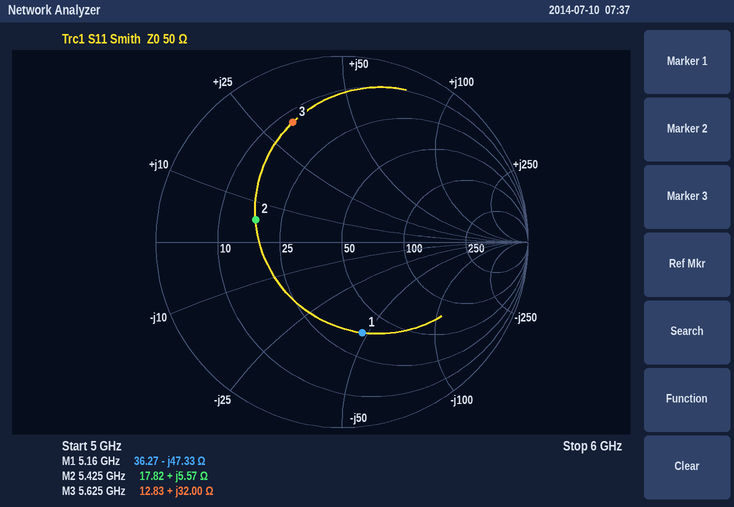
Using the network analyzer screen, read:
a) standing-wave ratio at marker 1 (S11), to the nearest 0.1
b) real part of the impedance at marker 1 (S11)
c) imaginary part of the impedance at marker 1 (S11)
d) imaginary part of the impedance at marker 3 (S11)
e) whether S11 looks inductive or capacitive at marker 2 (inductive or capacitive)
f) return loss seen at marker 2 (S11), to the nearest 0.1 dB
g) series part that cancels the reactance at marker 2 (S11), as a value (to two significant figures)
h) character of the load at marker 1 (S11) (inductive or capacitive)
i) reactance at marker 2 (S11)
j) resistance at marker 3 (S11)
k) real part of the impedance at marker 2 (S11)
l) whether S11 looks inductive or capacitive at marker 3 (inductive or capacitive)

3.0
36.27 Ω
-47.33 Ω
+32.00 Ω
inductive
6.4 dB
5.3 pF
capacitive
+5.57 Ω
12.83 Ω
17.82 Ω
inductive
